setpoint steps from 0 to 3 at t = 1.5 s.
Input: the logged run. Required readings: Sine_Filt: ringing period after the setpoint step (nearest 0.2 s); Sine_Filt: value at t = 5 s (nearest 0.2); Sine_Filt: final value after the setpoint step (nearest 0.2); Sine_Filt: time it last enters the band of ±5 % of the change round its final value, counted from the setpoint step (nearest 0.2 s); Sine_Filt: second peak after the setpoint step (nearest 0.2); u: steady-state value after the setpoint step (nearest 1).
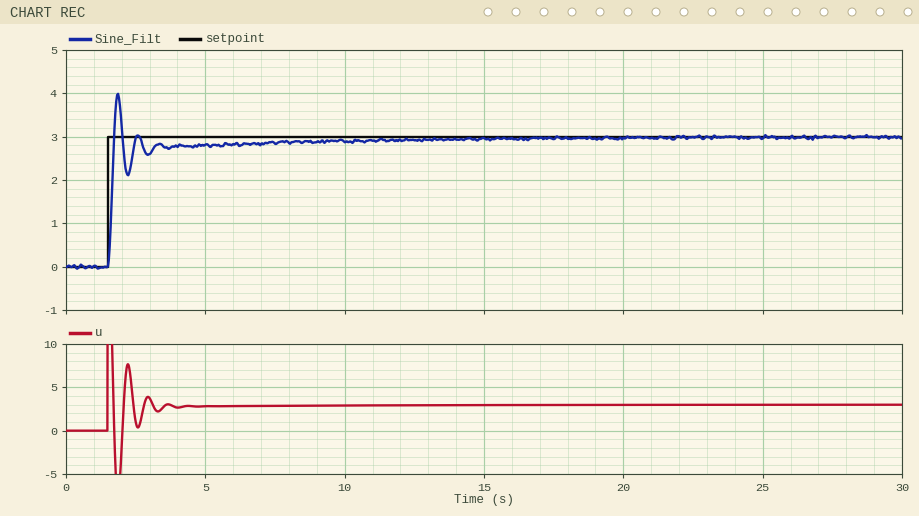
0.8 s
2.8
3.0
5.6 s
3.0
3
